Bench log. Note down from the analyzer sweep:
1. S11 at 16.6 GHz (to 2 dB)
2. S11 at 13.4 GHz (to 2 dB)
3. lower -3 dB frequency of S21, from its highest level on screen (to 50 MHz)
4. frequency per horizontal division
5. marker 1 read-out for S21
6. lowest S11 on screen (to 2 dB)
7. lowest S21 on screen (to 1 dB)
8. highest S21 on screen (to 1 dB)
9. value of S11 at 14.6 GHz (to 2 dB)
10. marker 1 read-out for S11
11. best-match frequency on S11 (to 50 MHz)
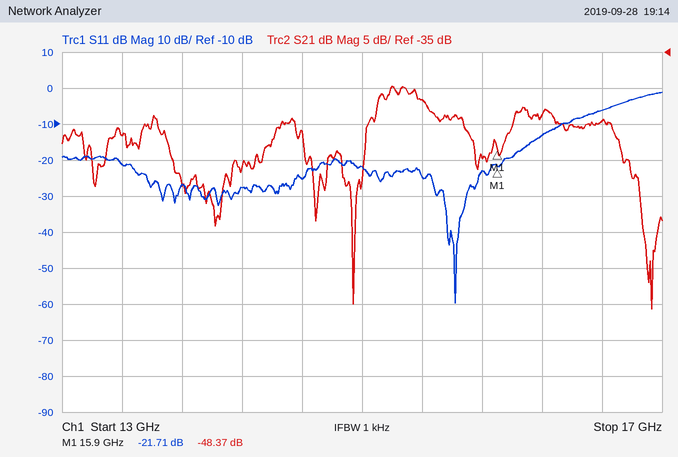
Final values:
-6 dB
-22 dB
15.10 GHz
400 MHz
-48.37 dB
-60 dB
-71 dB
-40 dB
-26 dB
-21.71 dB
15.60 GHz
